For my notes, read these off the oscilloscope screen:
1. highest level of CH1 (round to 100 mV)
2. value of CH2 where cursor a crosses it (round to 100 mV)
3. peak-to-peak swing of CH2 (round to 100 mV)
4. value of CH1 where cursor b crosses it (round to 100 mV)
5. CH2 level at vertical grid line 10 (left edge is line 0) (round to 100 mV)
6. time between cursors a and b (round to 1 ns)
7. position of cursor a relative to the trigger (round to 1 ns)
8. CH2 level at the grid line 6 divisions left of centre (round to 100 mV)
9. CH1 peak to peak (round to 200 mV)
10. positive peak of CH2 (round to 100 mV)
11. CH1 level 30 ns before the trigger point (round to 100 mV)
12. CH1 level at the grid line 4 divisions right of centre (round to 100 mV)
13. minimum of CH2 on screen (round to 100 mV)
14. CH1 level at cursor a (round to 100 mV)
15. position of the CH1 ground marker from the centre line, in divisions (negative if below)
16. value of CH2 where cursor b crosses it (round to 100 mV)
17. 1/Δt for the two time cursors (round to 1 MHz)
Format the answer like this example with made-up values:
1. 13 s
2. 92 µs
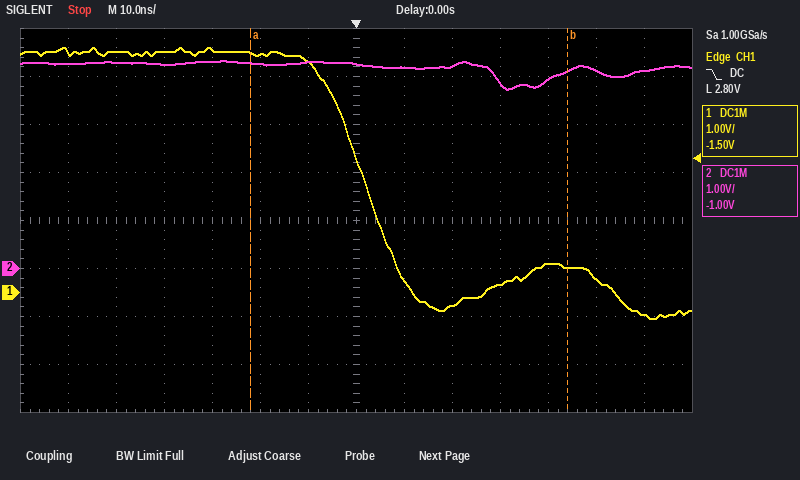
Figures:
1. 5.1 V
2. 4.3 V
3. 600 mV
4. 500 mV
5. 3.9 V
6. 66 ns
7. -22 ns
8. 4.3 V
9. 5.6 V
10. 4.3 V
11. 5.1 V
12. 600 mV
13. 3.7 V
14. 5.0 V
15. -1.5 div
16. 4.1 V
17. 15 MHz
